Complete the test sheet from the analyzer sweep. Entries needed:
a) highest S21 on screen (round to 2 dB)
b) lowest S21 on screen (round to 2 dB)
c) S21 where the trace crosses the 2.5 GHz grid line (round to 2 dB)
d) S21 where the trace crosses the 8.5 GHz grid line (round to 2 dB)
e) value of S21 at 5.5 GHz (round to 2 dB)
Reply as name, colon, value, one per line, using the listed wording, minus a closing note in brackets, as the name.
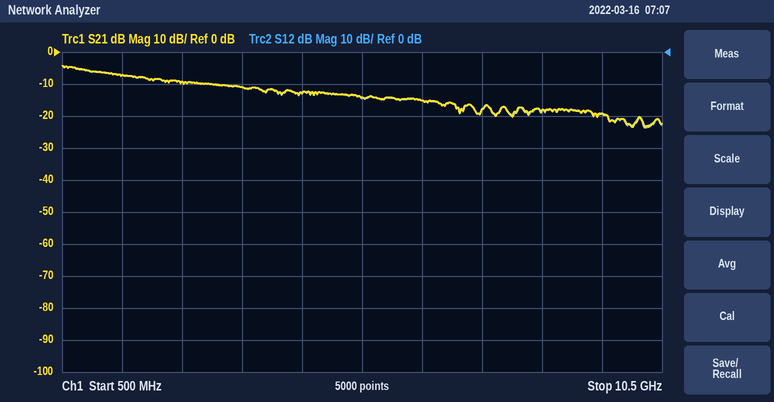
highest S21 on screen: -4 dB
lowest S21 on screen: -24 dB
S21 where the trace crosses the 2.5 GHz grid line: -10 dB
S21 where the trace crosses the 8.5 GHz grid line: -18 dB
value of S21 at 5.5 GHz: -14 dB
